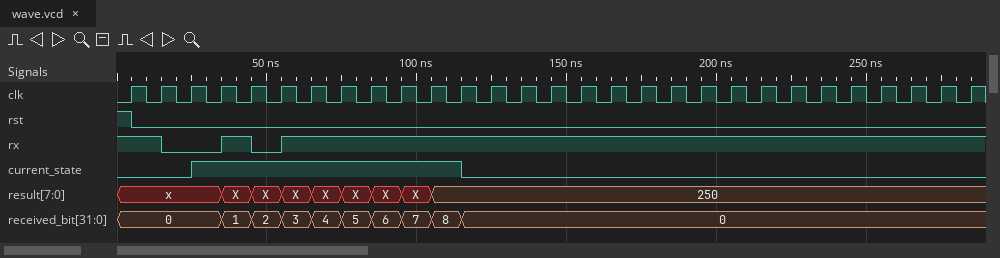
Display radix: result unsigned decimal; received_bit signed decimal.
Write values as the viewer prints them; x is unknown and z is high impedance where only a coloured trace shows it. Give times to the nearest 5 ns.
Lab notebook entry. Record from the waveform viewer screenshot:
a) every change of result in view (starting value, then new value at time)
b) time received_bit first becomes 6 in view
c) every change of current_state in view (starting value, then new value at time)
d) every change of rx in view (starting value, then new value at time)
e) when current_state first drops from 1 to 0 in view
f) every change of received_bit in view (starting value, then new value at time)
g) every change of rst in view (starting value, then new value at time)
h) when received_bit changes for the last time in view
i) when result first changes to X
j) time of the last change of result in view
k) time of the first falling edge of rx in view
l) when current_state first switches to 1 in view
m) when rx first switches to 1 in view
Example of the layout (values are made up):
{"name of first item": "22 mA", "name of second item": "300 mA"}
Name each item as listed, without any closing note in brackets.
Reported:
{"every change of result in view": "x, X at 35 ns, X at 45 ns, X at 55 ns, X at 65 ns, X at 75 ns, X at 85 ns, X at 95 ns, 250 at 105 ns", "time received_bit first becomes 6 in view": "85 ns", "every change of current_state in view": "0, 1 at 25 ns, 0 at 115 ns", "every change of rx in view": "1, 0 at 15 ns, 1 at 35 ns, 0 at 45 ns, 1 at 55 ns", "when current_state first drops from 1 to 0 in view": "115 ns", "every change of received_bit in view": "0, 1 at 35 ns, 2 at 45 ns, 3 at 55 ns, 4 at 65 ns, 5 at 75 ns, 6 at 85 ns, 7 at 95 ns, 8 at 105 ns, 0 at 115 ns", "every change of rst in view": "1, 0 at 5 ns", "when received_bit changes for the last time in view": "115 ns", "when result first changes to X": "35 ns", "time of the last change of result in view": "105 ns", "time of the first falling edge of rx in view": "15 ns", "when current_state first switches to 1 in view": "25 ns", "when rx first switches to 1 in view": "35 ns"}
